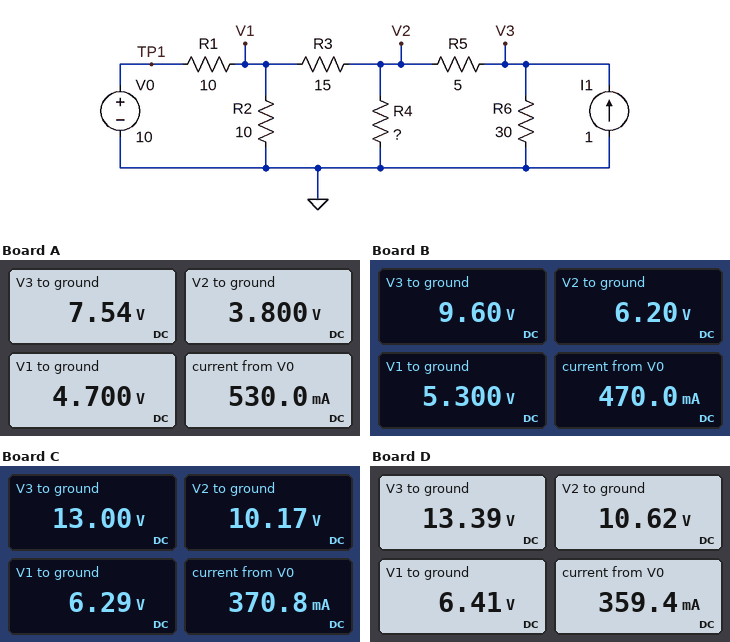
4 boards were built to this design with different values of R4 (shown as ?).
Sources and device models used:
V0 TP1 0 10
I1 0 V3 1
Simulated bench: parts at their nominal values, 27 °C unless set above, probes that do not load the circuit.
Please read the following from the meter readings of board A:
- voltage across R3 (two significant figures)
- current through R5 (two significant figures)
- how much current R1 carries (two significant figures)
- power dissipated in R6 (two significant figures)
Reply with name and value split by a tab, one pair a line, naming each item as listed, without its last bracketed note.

voltage across R3	900 mV
current through R5	750 mA
how much current R1 carries	530 mA
power dissipated in R6	1.9 W
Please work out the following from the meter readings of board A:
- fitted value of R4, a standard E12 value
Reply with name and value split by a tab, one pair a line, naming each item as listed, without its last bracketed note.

fitted value of R4, a standard E12 value	4.7 Ω
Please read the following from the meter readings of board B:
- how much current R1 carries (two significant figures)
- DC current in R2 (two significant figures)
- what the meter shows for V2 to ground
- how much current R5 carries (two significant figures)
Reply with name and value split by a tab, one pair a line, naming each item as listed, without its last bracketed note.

how much current R1 carries	470 mA
DC current in R2	530 mA
what the meter shows for V2 to ground	6.20 V
how much current R5 carries	680 mA
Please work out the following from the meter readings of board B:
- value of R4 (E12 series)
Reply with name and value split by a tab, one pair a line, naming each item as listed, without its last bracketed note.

value of R4	10 Ω
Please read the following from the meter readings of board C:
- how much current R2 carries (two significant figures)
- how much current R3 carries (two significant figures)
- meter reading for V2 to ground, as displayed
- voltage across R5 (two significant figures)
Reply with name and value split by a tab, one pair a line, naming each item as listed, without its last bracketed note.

how much current R2 carries	630 mA
how much current R3 carries	260 mA
meter reading for V2 to ground, as displayed	10.17 V
voltage across R5	2.8 V
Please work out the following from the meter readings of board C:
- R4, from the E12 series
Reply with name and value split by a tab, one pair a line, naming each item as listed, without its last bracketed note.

R4, from the E12 series	33 Ω
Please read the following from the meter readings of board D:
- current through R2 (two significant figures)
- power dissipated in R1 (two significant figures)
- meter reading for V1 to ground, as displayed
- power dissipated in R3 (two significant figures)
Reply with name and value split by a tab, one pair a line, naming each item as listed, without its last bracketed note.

current through R2	640 mA
power dissipated in R1	1.3 W
meter reading for V1 to ground, as displayed	6.41 V
power dissipated in R3	1.2 W
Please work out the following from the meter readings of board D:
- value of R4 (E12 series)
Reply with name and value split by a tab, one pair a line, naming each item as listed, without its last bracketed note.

value of R4	39 Ω
